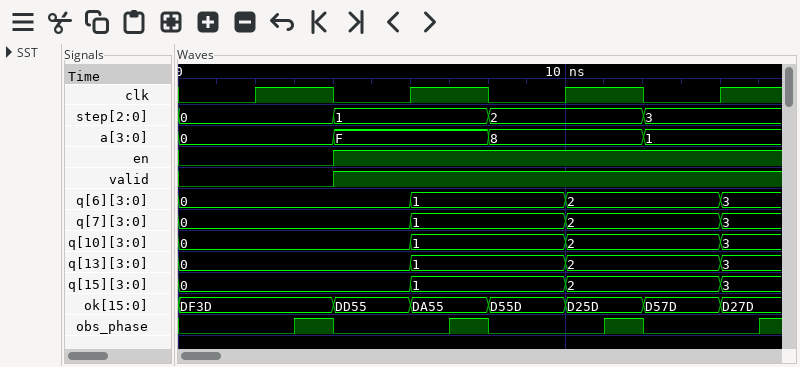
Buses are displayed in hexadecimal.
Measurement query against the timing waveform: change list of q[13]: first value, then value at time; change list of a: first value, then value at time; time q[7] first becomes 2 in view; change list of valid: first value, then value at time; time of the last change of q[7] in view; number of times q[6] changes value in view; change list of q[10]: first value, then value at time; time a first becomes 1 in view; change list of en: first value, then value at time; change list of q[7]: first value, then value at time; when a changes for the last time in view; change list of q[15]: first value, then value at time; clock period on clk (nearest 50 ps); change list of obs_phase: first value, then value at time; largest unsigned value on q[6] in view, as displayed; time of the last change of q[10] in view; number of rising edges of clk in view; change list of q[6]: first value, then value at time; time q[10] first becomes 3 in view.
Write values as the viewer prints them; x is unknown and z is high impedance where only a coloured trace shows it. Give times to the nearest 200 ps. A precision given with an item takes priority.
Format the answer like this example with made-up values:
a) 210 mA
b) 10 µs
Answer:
a) 0, 1 at 6000 ps, 2 at 10000 ps, 3 at 14000 ps
b) 0, F at 4000 ps, 8 at 8000 ps, 1 at 12000 ps
c) 10000 ps
d) 0, 1 at 4000 ps
e) 14000 ps
f) 3
g) 0, 1 at 6000 ps, 2 at 10000 ps, 3 at 14000 ps
h) 12000 ps
i) 0, 1 at 4000 ps
j) 0, 1 at 6000 ps, 2 at 10000 ps, 3 at 14000 ps
k) 12000 ps
l) 0, 1 at 6000 ps, 2 at 10000 ps, 3 at 14000 ps
m) 4000 ps
n) 0, 1 at 3000 ps, 0 at 4000 ps, 1 at 7000 ps, 0 at 8000 ps, 1 at 11000 ps, 0 at 12000 ps, 1 at 15000 ps
o) 3
p) 14000 ps
q) 4
r) 0, 1 at 6000 ps, 2 at 10000 ps, 3 at 14000 ps
s) 14000 ps
